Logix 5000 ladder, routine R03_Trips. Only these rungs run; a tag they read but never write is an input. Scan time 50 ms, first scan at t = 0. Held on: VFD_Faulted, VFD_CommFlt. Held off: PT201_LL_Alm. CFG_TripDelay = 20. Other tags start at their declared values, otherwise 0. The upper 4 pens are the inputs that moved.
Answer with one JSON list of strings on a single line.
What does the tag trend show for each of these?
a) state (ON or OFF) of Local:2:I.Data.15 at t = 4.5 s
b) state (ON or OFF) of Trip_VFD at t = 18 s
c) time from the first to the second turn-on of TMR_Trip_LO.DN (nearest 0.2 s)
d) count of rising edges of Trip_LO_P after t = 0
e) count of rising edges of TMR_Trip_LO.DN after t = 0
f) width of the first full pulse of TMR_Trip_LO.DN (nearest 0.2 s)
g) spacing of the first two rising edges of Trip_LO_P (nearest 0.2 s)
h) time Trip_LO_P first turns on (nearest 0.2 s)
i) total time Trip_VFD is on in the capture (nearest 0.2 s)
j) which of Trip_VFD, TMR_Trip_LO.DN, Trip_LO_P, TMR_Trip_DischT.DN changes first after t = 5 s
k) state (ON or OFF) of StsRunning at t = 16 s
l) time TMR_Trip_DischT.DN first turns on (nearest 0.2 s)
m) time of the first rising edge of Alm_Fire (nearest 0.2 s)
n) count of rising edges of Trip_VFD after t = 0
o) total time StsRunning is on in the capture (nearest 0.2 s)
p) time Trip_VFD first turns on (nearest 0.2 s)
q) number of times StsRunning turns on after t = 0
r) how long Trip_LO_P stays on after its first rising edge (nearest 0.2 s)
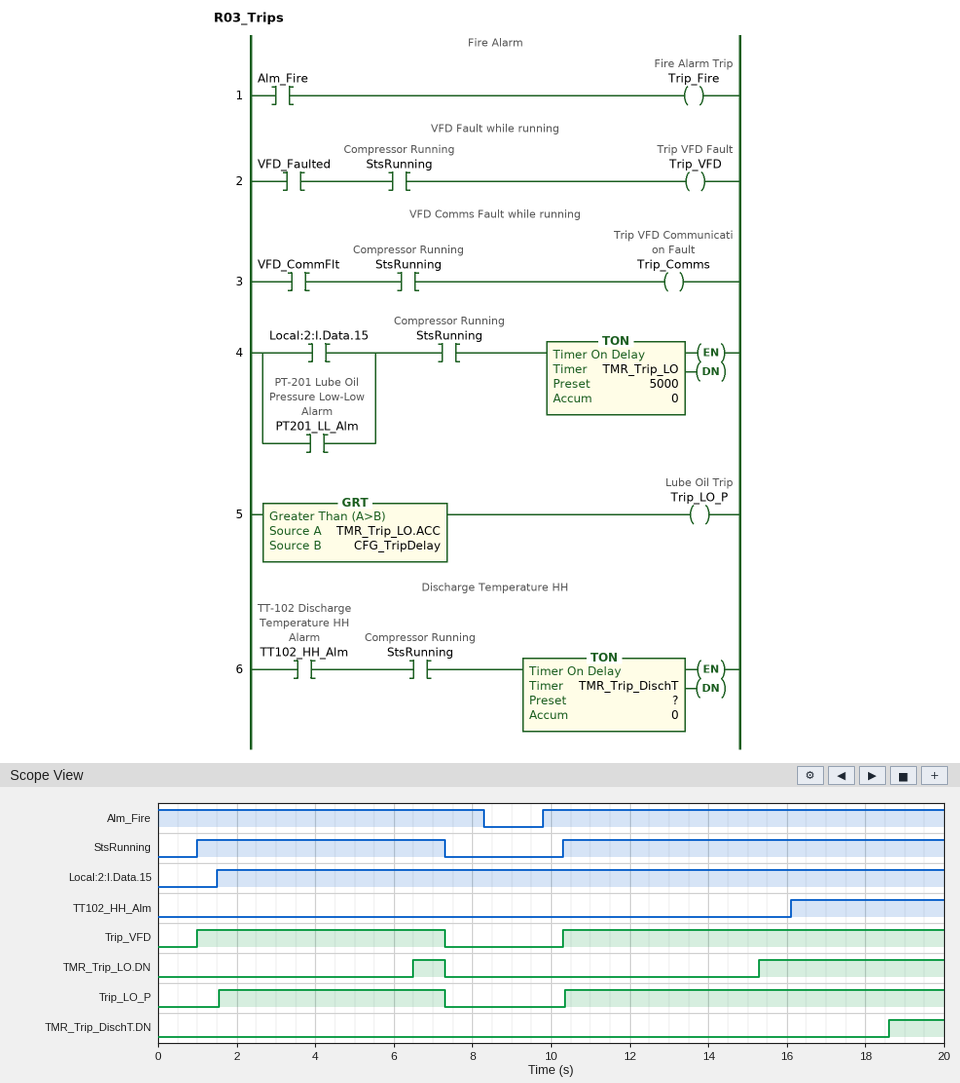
["ON", "ON", "8.8 s", "2", "2", "0.8 s", "8.8 s", "1.6 s", "16.0 s", "TMR_Trip_LO.DN", "ON", "18.6 s", "9.8 s", "2", "16.0 s", "1.0 s", "2", "5.8 s"]
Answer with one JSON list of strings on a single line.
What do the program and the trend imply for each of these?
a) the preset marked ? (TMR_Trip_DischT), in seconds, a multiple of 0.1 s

["2.5 s"]
